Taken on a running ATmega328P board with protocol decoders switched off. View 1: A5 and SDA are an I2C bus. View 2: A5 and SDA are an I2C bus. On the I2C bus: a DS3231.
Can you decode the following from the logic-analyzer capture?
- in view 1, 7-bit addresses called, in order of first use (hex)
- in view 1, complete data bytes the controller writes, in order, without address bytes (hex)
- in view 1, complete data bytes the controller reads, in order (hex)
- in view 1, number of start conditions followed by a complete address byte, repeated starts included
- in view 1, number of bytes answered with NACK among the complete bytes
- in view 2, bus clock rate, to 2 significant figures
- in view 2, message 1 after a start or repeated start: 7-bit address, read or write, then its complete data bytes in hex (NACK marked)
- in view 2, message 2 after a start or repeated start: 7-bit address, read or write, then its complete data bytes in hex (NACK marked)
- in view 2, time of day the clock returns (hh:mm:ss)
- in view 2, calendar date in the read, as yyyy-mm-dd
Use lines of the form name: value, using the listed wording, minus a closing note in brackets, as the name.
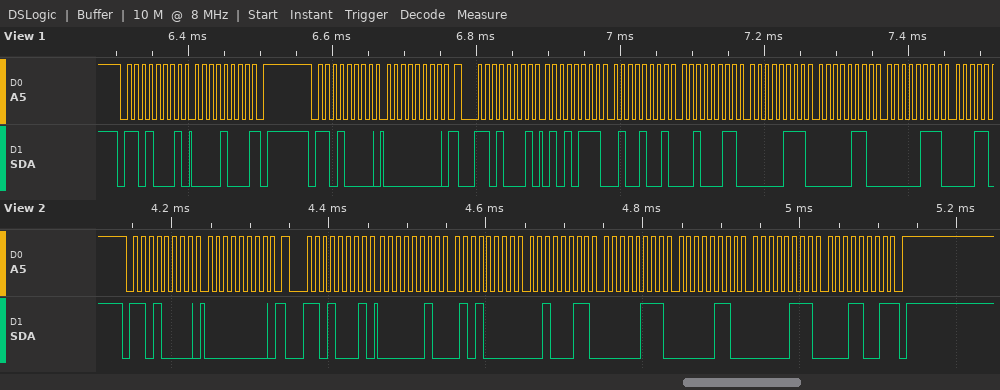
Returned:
in view 1, 7-bit addresses called, in order of first use: 0x68
in view 1, complete data bytes the controller writes, in order, without address bytes: 00
in view 1, complete data bytes the controller reads, in order: 08 57 49 23 07 06 07
in view 1, number of start conditions followed by a complete address byte, repeated starts included: 3
in view 1, number of bytes answered with NACK among the complete bytes: 1
in view 2, bus clock rate, to 2 significant figures: 100 kHz
in view 2, message 1 after a start or repeated start: 7-bit address, read or write, then its complete data bytes in hex: 0x68 write: 00
in view 2, message 2 after a start or repeated start: 7-bit address, read or write, then its complete data bytes in hex: 0x68 read: 02 50 23 07 06 07 19 NACK
in view 2, time of day the clock returns: 23:50:02
in view 2, calendar date in the read, as yyyy-mm-dd: 2019-07-06
